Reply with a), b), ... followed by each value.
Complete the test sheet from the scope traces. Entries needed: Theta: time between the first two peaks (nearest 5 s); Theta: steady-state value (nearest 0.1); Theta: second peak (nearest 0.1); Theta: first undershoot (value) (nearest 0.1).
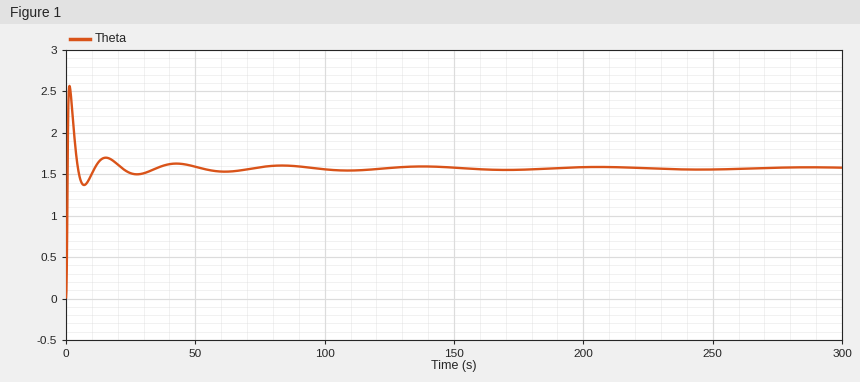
a) 15 s
b) 1.6
c) 1.7
d) 1.4
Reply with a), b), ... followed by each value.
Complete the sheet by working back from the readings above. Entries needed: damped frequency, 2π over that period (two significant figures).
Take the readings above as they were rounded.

a) 0.42 rad/s
